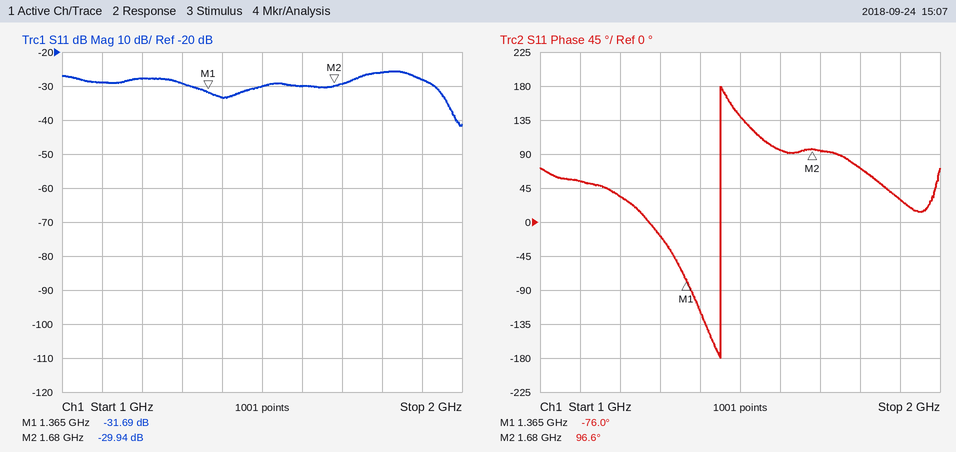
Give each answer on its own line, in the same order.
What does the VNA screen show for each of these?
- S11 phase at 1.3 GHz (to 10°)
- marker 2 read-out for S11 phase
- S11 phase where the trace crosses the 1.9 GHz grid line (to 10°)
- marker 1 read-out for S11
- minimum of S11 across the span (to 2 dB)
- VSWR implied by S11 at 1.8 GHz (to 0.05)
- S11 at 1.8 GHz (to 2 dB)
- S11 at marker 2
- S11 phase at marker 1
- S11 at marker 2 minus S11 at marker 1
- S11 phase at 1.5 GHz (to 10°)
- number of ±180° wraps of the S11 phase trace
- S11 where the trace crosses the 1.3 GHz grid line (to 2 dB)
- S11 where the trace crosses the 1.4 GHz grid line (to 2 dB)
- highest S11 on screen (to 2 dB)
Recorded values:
-20°
96.6°
30°
-31.69 dB
-42 dB
1.10
-26 dB
-29.94 dB
-76.0°
1.75 dB
140°
1
-30 dB
-34 dB
-26 dB
